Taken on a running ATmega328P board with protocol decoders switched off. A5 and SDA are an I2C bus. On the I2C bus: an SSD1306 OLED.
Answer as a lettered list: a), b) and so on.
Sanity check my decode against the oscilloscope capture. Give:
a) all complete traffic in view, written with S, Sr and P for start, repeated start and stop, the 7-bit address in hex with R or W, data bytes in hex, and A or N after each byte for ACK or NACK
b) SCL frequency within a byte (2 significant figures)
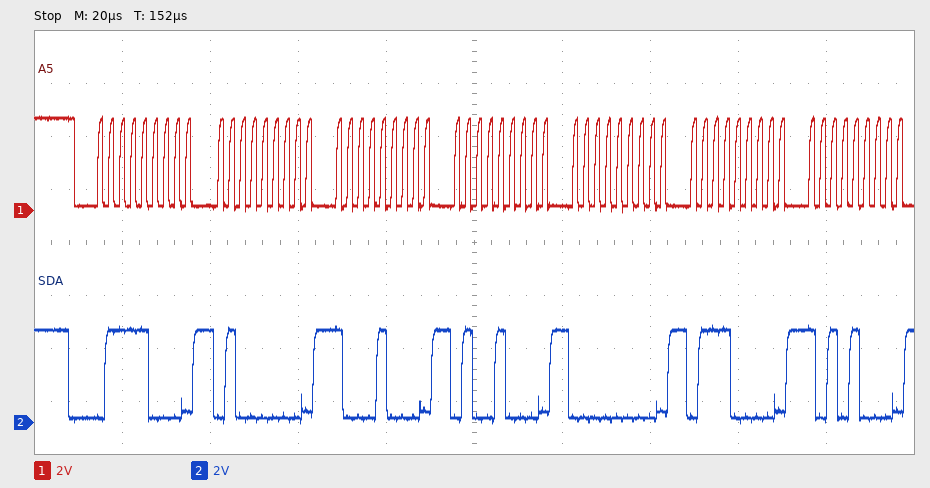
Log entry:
a) S 3CW A 40 A 88 A 48 A 00 A 70 A A8 A
b) 400 kHz
